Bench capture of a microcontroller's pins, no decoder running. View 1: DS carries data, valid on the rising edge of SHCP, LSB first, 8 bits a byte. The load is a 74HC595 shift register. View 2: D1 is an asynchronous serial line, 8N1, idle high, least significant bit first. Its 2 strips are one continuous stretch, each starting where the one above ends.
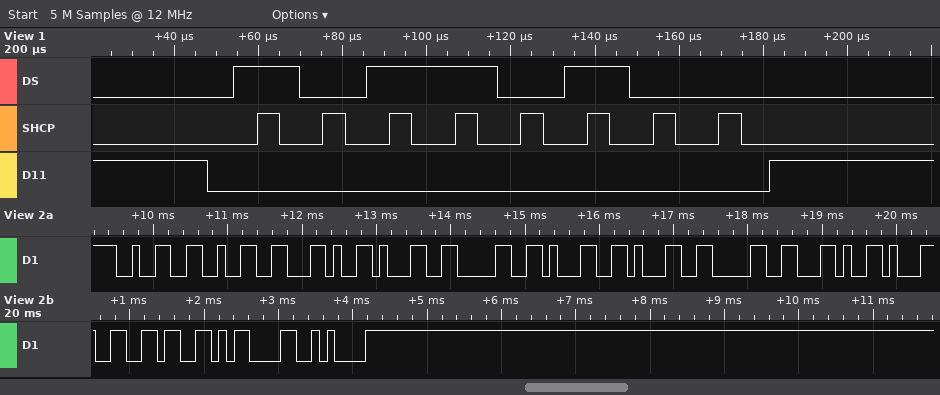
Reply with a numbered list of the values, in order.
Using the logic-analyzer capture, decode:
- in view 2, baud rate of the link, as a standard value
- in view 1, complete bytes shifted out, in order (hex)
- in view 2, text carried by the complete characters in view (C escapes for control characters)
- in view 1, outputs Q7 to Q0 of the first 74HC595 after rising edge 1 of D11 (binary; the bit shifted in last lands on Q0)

1. 9600 baud
2. 2D
3. "22,10110,16\r\n"
4. 10110100
